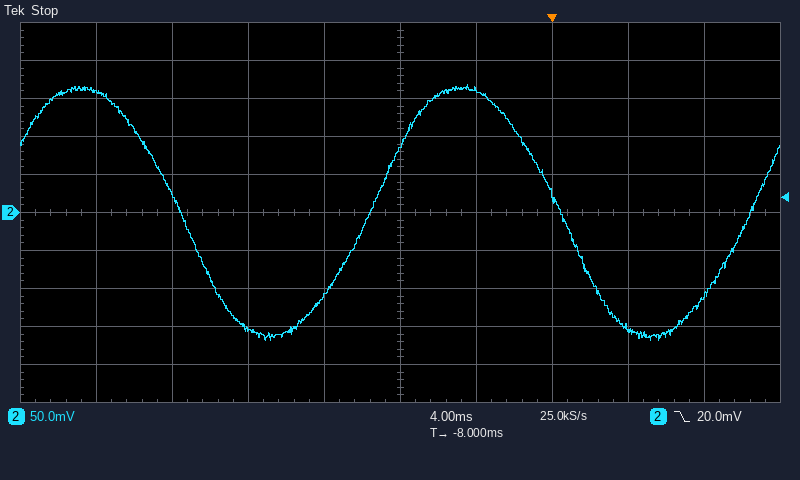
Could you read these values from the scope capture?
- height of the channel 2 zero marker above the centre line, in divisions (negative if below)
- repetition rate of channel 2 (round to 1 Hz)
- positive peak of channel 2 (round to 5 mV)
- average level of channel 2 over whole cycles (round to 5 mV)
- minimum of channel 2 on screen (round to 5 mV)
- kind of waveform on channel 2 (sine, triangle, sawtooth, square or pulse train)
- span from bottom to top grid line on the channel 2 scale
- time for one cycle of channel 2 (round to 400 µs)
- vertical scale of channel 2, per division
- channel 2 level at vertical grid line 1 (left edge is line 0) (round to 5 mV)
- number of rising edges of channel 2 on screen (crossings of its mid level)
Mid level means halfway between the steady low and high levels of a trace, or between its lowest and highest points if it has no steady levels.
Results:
0.0 div
50 Hz
170 mV
0 mV
-170 mV
sine
500 mV
20.0 ms
50 mV
160 mV
2
